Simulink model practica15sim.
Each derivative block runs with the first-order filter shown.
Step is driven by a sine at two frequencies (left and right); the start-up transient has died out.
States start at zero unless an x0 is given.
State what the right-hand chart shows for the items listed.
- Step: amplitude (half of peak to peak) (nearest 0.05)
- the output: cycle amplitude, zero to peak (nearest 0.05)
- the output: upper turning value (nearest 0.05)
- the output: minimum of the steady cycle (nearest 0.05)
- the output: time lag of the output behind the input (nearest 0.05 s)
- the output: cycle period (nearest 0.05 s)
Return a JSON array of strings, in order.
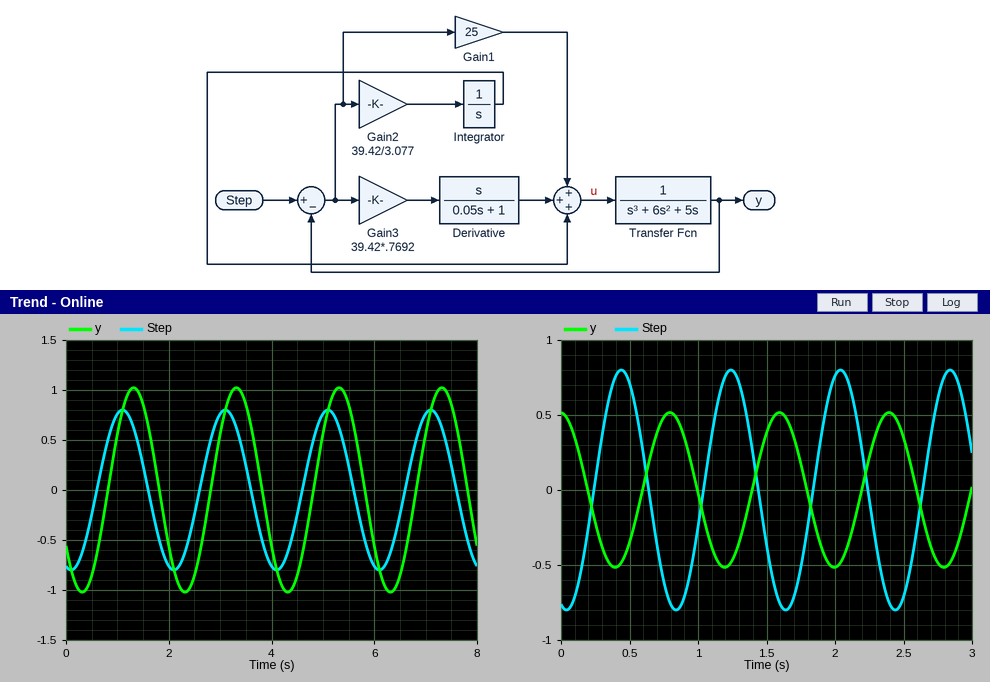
["0.80", "0.50", "0.50", "-0.50", "0.35 s", "0.80 s"]
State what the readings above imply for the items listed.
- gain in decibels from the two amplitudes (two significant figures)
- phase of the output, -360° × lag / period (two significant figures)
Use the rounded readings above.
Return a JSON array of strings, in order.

["-4.1 dB", "-160°"]
